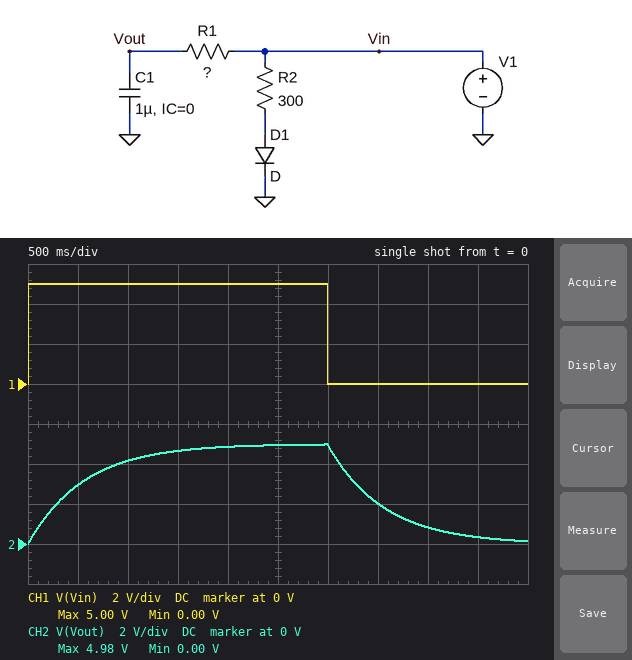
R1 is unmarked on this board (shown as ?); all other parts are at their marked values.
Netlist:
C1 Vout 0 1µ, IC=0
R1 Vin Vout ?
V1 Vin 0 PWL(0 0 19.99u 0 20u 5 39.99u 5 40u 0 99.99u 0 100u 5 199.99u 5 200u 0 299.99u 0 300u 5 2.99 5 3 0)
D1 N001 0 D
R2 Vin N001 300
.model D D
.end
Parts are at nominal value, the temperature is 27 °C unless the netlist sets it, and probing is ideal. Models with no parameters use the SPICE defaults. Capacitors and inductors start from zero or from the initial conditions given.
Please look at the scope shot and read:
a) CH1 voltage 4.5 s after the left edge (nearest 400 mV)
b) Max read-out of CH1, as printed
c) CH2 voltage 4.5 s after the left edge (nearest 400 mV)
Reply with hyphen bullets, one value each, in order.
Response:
- 0 V
- 5.00 V
- 400 mV
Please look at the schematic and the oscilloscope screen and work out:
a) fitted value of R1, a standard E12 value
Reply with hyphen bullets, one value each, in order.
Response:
- 560 kΩ
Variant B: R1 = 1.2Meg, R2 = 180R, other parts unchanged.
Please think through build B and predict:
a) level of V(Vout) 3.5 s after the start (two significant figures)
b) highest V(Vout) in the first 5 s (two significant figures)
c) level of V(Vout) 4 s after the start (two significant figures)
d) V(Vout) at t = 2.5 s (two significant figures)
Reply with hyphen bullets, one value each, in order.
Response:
- 3.0 V
- 4.6 V
- 2.0 V
- 4.4 V
